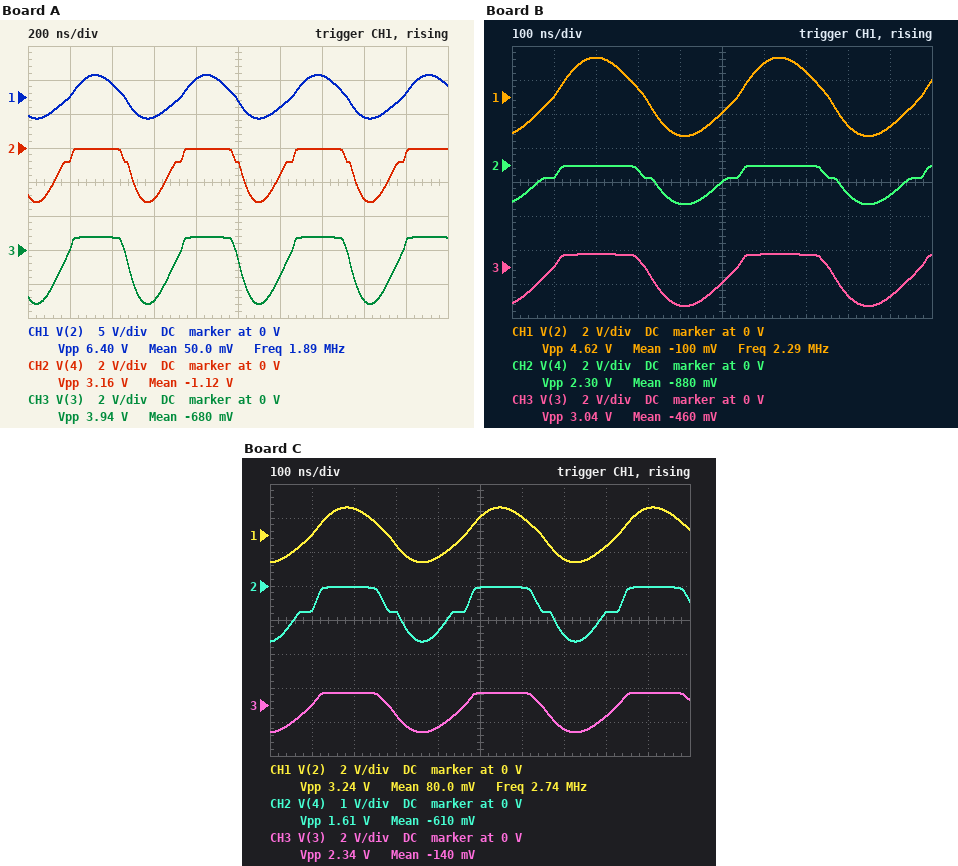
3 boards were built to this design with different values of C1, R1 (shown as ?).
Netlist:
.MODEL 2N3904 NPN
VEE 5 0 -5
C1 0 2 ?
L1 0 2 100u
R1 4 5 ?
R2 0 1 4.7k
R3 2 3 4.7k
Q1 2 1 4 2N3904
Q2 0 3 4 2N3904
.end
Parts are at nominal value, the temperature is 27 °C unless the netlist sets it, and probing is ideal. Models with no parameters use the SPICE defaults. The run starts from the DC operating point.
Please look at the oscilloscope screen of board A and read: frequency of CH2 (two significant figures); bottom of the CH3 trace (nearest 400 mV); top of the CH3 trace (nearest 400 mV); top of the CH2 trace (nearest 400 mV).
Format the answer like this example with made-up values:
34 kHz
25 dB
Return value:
1.9 MHz
-3.2 V
800 mV
0 V
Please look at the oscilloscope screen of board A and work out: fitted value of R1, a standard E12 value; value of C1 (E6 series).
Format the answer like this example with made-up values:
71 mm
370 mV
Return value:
3.3 kΩ
68 pF
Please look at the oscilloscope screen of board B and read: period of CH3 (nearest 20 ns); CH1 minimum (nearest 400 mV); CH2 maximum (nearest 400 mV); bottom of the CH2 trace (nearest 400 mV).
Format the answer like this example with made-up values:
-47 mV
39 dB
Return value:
440 ns
-2.4 V
0 V
-2.4 V
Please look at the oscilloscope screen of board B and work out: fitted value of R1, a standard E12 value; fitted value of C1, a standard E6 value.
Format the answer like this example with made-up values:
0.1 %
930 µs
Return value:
6.8 kΩ
47 pF
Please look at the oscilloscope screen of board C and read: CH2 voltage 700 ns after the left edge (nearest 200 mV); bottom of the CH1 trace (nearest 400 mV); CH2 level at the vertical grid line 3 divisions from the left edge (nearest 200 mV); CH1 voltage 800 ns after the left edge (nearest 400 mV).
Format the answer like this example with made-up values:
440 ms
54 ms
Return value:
-1.4 V
-1.6 V
-800 mV
-800 mV
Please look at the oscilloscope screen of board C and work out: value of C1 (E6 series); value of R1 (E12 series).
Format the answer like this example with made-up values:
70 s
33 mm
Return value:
33 pF
15 kΩ
